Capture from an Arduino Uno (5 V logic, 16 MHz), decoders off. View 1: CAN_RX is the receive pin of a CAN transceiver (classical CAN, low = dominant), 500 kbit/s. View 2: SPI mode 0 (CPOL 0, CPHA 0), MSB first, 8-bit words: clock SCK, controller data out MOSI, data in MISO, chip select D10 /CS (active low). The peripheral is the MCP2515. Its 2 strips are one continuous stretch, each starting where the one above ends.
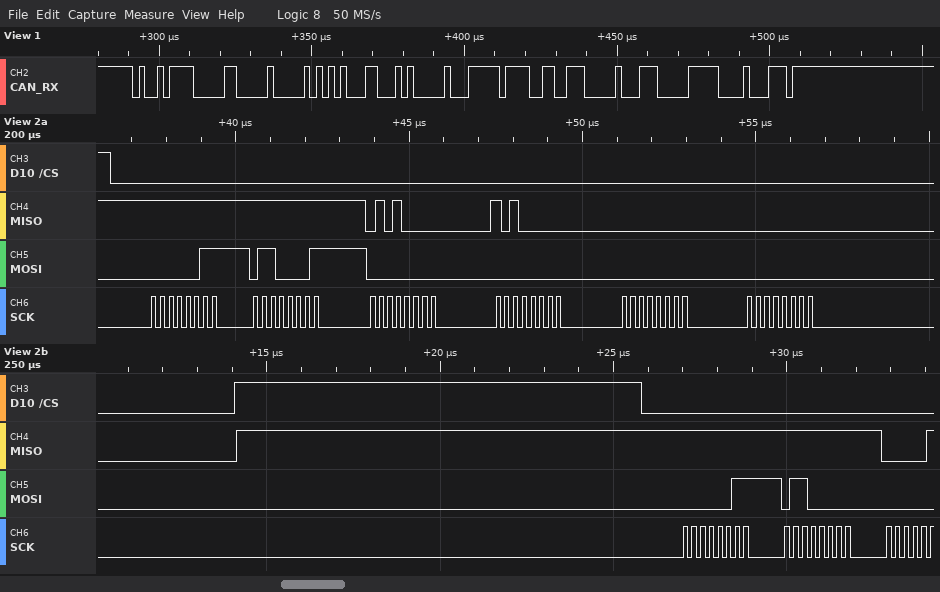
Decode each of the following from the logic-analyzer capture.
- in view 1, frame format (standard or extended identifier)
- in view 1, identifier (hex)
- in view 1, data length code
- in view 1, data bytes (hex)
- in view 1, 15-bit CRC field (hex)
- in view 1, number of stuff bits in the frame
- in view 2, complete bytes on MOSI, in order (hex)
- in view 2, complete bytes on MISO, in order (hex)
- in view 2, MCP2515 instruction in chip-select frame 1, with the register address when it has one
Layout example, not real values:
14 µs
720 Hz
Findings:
standard
0x4BC
8
00 A8 C5 00 FF 99 C0 38
0x1E23
8
03 61 00 00 00 00 03 60
FF FF 50 A0 00 00 FF FF
READ 0x61
